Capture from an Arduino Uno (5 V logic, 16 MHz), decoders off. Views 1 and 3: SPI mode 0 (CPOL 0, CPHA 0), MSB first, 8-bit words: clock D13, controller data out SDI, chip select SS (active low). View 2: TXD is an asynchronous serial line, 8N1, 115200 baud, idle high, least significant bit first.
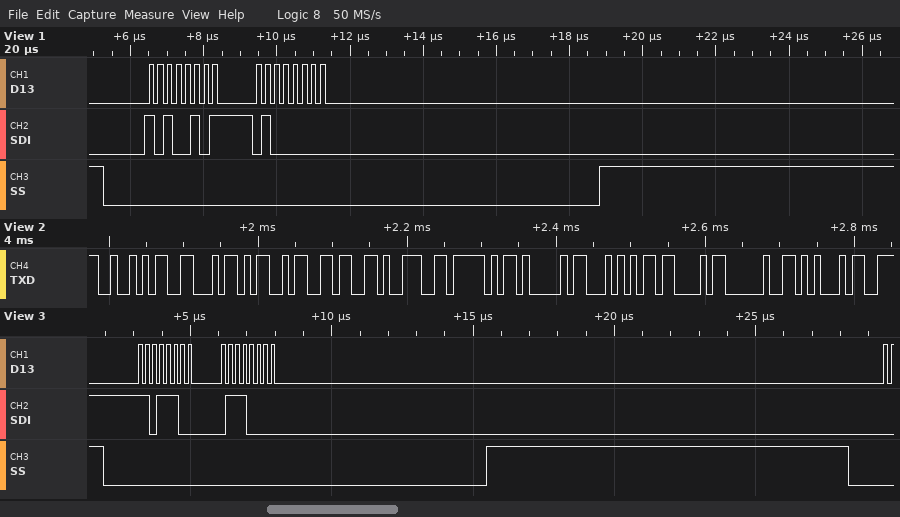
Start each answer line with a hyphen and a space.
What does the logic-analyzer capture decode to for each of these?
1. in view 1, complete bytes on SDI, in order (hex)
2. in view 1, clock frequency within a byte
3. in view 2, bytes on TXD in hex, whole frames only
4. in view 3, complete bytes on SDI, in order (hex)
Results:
- A5 40
- 4 MHz
- 52 46 4D 36 39 5F 41 54 43 20 45
- DC 70
